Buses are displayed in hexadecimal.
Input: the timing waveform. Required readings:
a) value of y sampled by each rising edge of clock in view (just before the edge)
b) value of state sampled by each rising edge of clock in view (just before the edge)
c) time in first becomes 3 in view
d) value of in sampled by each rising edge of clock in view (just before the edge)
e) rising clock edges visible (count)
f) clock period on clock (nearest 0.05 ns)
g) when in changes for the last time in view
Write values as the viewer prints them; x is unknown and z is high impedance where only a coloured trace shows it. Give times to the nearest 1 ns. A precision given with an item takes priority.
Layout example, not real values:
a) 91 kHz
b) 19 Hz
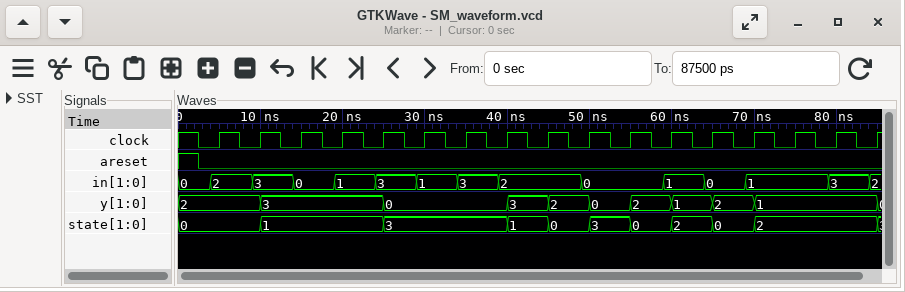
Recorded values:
a) 2, 2, 3, 3, 3, 0, 0, 0, 3, 2, 0, 2, 1, 2, 1, 1, 1
b) 0, 0, 1, 1, 1, 3, 3, 3, 1, 0, 3, 0, 2, 0, 2, 2, 2
c) 9 ns
d) 2, 3, 0, 1, 3, 1, 3, 2, 2, 0, 0, 1, 0, 1, 1, 3, 2
e) 17
f) 5 ns
g) 84 ns
